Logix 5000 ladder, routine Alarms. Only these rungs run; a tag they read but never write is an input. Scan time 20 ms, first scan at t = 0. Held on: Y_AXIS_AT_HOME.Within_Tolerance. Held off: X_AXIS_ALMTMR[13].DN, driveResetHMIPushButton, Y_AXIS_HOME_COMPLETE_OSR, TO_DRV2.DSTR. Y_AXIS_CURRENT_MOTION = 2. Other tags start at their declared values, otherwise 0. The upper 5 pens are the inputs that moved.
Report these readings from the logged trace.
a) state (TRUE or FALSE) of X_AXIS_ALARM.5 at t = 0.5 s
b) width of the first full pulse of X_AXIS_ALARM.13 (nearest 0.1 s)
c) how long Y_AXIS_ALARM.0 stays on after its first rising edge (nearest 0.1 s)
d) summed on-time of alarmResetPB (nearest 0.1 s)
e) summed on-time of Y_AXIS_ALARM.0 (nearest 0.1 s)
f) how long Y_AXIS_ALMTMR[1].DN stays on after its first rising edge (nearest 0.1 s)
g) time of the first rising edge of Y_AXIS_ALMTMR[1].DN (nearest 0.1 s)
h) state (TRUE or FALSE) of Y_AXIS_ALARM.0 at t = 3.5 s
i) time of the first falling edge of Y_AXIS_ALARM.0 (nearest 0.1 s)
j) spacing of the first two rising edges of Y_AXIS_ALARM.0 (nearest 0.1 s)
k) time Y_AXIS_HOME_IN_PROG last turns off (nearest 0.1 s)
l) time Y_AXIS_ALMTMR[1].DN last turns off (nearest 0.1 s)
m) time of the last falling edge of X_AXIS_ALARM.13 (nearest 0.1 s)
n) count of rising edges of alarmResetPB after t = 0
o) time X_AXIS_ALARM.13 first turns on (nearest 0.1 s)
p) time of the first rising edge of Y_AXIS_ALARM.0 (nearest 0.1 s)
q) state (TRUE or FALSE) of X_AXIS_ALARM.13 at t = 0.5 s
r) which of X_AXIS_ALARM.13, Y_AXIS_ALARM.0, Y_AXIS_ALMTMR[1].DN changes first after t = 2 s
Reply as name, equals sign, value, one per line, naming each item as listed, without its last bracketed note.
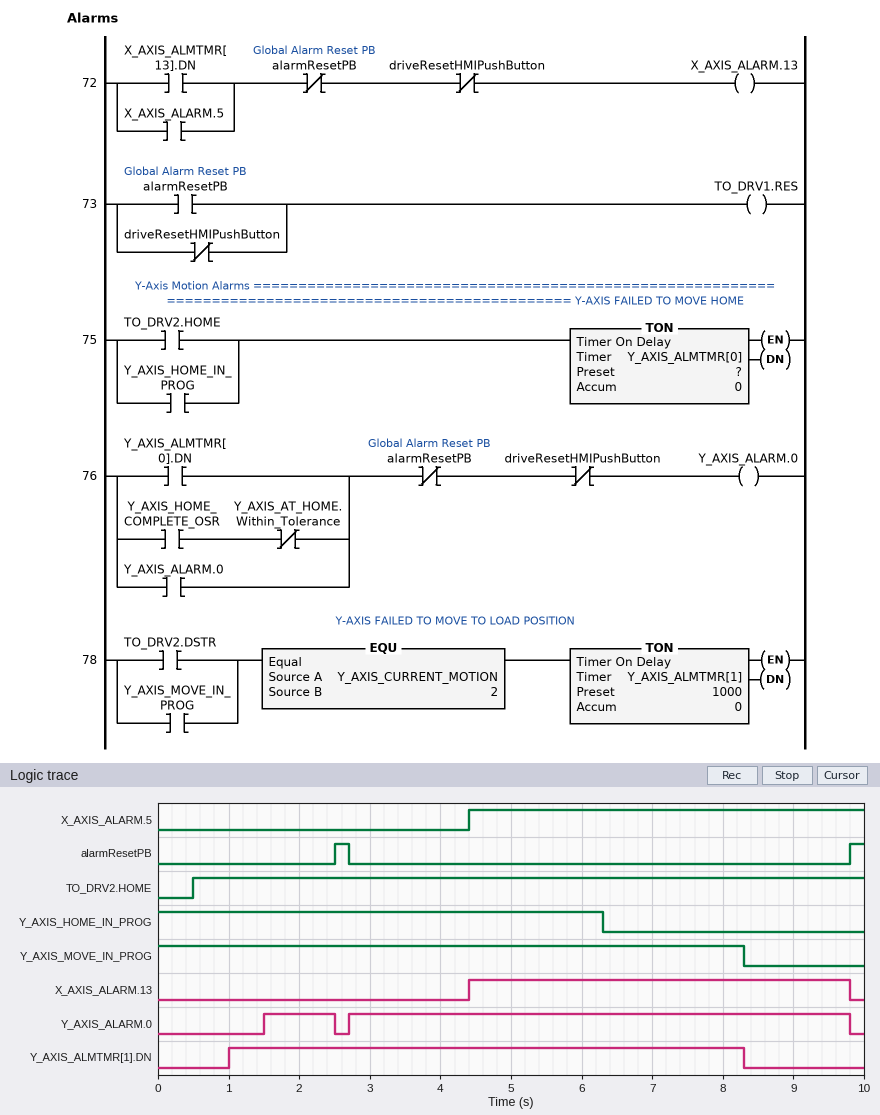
state (TRUE or FALSE) of X_AXIS_ALARM.5 at t = 0.5 s = FALSE
width of the first full pulse of X_AXIS_ALARM.13 = 5.4 s
how long Y_AXIS_ALARM.0 stays on after its first rising edge = 1.0 s
summed on-time of alarmResetPB = 0.4 s
summed on-time of Y_AXIS_ALARM.0 = 8.1 s
how long Y_AXIS_ALMTMR[1].DN stays on after its first rising edge = 7.3 s
time of the first rising edge of Y_AXIS_ALMTMR[1].DN = 1.0 s
state (TRUE or FALSE) of Y_AXIS_ALARM.0 at t = 3.5 s = TRUE
time of the first falling edge of Y_AXIS_ALARM.0 = 2.5 s
spacing of the first two rising edges of Y_AXIS_ALARM.0 = 1.2 s
time Y_AXIS_HOME_IN_PROG last turns off = 6.3 s
time Y_AXIS_ALMTMR[1].DN last turns off = 8.3 s
time of the last falling edge of X_AXIS_ALARM.13 = 9.8 s
count of rising edges of alarmResetPB after t = 0 = 2
time X_AXIS_ALARM.13 first turns on = 4.4 s
time of the first rising edge of Y_AXIS_ALARM.0 = 1.5 s
state (TRUE or FALSE) of X_AXIS_ALARM.13 at t = 0.5 s = FALSE
which of X_AXIS_ALARM.13, Y_AXIS_ALARM.0, Y_AXIS_ALMTMR[1].DN changes first after t = 2 s = Y_AXIS_ALARM.0
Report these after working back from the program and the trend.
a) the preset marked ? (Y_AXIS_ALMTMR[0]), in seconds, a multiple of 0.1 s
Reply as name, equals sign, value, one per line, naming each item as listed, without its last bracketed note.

the preset marked ? (Y_AXIS_ALMTMR[0]), in seconds, a multiple of 0.1 s = 1.5 s
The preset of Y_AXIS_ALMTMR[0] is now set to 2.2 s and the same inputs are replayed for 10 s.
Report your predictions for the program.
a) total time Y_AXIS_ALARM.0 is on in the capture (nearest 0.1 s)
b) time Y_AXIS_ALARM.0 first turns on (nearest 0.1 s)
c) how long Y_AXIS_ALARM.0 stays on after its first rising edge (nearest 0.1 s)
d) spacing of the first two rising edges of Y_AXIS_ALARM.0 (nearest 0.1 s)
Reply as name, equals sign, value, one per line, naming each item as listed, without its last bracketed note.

total time Y_AXIS_ALARM.0 is on in the capture = 7.4 s
time Y_AXIS_ALARM.0 first turns on = 2.2 s
how long Y_AXIS_ALARM.0 stays on after its first rising edge = 0.3 s
spacing of the first two rising edges of Y_AXIS_ALARM.0 = 0.5 s
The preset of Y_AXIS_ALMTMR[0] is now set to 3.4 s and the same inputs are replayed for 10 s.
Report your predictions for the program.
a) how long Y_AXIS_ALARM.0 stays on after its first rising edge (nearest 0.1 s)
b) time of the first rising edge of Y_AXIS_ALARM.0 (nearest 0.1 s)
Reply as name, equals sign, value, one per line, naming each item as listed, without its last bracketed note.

how long Y_AXIS_ALARM.0 stays on after its first rising edge = 6.4 s
time of the first rising edge of Y_AXIS_ALARM.0 = 3.4 s
